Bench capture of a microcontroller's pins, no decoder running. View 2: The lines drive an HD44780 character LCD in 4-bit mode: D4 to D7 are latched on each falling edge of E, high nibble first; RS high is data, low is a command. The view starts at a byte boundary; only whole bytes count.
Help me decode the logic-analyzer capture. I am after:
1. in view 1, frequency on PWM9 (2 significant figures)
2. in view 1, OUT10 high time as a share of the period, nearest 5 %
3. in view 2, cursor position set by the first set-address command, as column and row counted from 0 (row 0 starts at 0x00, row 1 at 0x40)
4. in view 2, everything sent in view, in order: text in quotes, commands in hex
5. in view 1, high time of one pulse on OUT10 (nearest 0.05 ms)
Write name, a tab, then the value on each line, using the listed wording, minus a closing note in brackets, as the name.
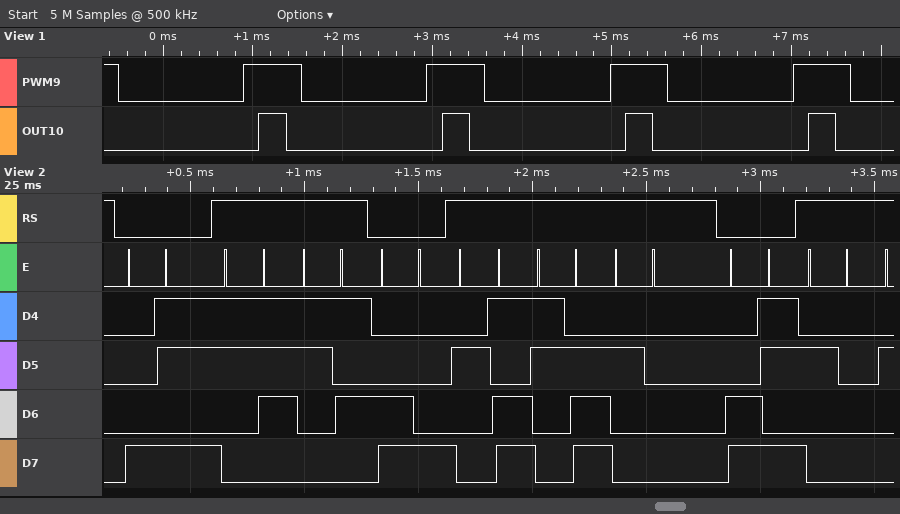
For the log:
in view 1, frequency on PWM9	490 Hz
in view 1, OUT10 high time as a share of the period, nearest 5 %	15 %
in view 2, cursor position set by the first set-address command, as column and row counted from 0	column 11, row 0
in view 2, everything sent in view, in order: text in quotes, commands in hex	0x8B "75" 0xC8 "-> " 0xCB " "
in view 1, high time of one pulse on OUT10	0.30 ms
